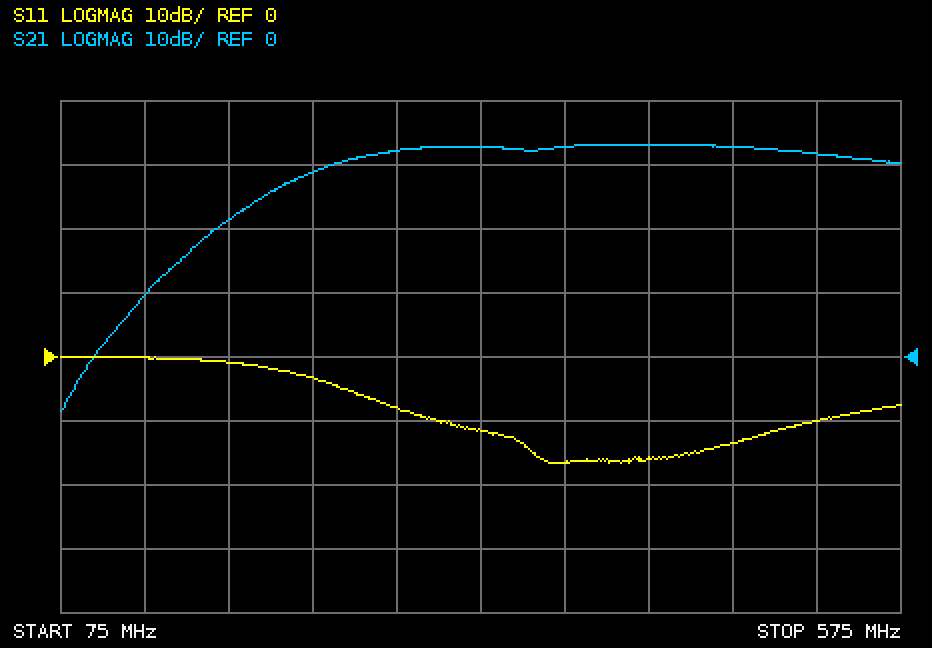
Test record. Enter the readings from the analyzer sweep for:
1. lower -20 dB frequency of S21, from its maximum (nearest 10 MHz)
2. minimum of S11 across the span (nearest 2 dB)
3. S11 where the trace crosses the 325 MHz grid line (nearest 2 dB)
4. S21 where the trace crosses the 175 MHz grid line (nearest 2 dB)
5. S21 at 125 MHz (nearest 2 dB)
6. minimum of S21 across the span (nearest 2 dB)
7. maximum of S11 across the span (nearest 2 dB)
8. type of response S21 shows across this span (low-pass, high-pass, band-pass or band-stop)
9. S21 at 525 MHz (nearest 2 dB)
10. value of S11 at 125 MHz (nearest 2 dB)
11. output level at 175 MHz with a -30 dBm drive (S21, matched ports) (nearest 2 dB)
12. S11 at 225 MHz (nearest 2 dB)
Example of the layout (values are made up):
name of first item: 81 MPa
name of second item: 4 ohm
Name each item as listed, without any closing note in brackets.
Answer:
lower -20 dB frequency of S21, from its maximum: 140 MHz
minimum of S11 across the span: -16 dB
S11 where the trace crosses the 325 MHz grid line: -12 dB
S21 where the trace crosses the 175 MHz grid line: 22 dB
S21 at 125 MHz: 10 dB
minimum of S21 across the span: -8 dB
maximum of S11 across the span: 0 dB
type of response S21 shows across this span: high-pass
S21 at 525 MHz: 32 dB
value of S11 at 125 MHz: 0 dB
output level at 175 MHz with a -30 dBm drive (S21, matched ports): -8 dBm
S11 at 225 MHz: -4 dB
